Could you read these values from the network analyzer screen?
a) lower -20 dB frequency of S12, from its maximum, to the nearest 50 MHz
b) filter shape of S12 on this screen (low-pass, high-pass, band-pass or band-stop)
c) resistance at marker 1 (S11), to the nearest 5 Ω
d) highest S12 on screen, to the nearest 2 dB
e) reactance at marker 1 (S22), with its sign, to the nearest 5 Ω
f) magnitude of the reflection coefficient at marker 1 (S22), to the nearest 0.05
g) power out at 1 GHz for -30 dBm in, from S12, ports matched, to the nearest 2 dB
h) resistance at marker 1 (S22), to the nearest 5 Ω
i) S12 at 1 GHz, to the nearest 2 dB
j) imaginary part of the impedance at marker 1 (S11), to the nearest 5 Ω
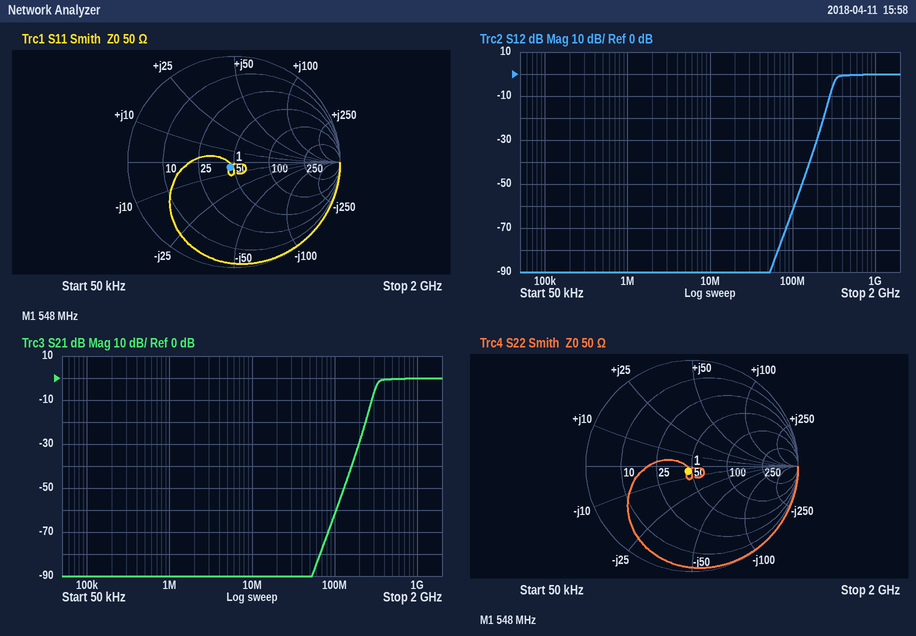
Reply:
250 MHz
high-pass
45 Ω
0 dB
-5 Ω
0.05
-30 dBm
45 Ω
0 dB
-5 Ω
